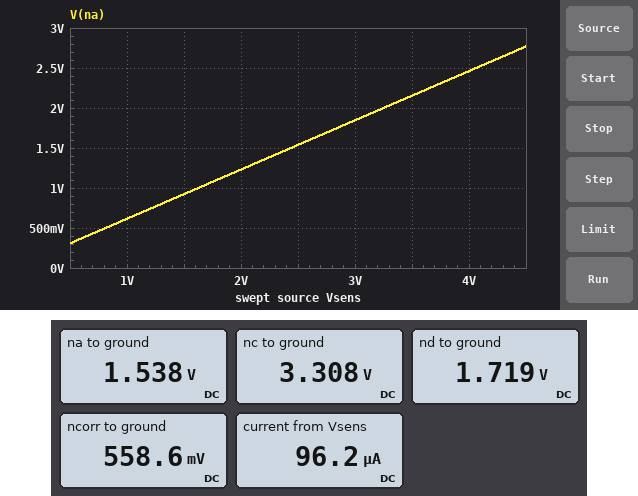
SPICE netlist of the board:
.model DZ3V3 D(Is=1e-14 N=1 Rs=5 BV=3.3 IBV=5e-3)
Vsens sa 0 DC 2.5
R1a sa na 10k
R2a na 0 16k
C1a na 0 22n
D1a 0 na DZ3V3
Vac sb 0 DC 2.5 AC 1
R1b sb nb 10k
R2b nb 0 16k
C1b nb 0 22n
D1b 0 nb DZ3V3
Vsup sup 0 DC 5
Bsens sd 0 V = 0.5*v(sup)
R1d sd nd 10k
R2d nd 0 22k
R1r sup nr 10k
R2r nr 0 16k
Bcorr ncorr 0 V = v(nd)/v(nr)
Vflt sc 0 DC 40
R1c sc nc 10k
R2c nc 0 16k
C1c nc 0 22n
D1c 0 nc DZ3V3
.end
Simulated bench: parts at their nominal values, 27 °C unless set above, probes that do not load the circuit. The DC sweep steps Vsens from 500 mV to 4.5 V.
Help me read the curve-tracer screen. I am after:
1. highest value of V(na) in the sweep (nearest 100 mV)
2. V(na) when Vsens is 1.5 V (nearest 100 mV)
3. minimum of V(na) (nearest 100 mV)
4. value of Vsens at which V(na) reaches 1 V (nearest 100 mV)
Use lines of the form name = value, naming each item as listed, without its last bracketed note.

highest value of V(na) in the sweep = 2.8 V
V(na) when Vsens is 1.5 V = 900 mV
minimum of V(na) = 300 mV
value of Vsens at which V(na) reaches 1 V = 1.6 V
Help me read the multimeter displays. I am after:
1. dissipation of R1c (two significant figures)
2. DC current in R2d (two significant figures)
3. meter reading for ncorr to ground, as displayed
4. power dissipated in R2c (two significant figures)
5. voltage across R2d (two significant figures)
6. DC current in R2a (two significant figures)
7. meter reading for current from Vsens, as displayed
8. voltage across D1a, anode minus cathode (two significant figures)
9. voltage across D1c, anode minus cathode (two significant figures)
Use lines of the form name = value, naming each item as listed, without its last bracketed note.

dissipation of R1c = 130 mW
DC current in R2d = 78 µA
meter reading for ncorr to ground, as displayed = 558.6 mV
power dissipated in R2c = 680 µW
voltage across R2d = 1.7 V
DC current in R2a = 96 µA
meter reading for current from Vsens, as displayed = 96.2 µA
voltage across D1a, anode minus cathode = -1.5 V
voltage across D1c, anode minus cathode = -3.3 V
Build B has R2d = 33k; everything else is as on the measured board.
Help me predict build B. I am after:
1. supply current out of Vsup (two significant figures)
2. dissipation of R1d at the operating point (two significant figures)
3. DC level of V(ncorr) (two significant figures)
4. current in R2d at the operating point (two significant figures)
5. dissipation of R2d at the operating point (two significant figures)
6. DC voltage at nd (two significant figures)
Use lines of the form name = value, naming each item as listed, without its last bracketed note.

supply current out of Vsup = 190 µA
dissipation of R1d at the operating point = 34 µW
DC level of V(ncorr) = 620 mV
current in R2d at the operating point = 58 µA
dissipation of R2d at the operating point = 110 µW
DC voltage at nd = 1.9 V
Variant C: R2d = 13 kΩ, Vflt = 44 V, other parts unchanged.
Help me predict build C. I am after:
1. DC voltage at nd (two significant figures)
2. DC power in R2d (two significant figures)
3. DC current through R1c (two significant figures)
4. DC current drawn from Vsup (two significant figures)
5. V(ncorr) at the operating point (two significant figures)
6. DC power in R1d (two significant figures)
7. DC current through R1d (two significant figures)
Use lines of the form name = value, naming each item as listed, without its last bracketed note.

DC voltage at nd = 1.4 V
DC power in R2d = 150 µW
DC current through R1c = 4.1 mA
DC current drawn from Vsup = 190 µA
V(ncorr) at the operating point = 460 mV
DC power in R1d = 120 µW
DC current through R1d = 110 µA
